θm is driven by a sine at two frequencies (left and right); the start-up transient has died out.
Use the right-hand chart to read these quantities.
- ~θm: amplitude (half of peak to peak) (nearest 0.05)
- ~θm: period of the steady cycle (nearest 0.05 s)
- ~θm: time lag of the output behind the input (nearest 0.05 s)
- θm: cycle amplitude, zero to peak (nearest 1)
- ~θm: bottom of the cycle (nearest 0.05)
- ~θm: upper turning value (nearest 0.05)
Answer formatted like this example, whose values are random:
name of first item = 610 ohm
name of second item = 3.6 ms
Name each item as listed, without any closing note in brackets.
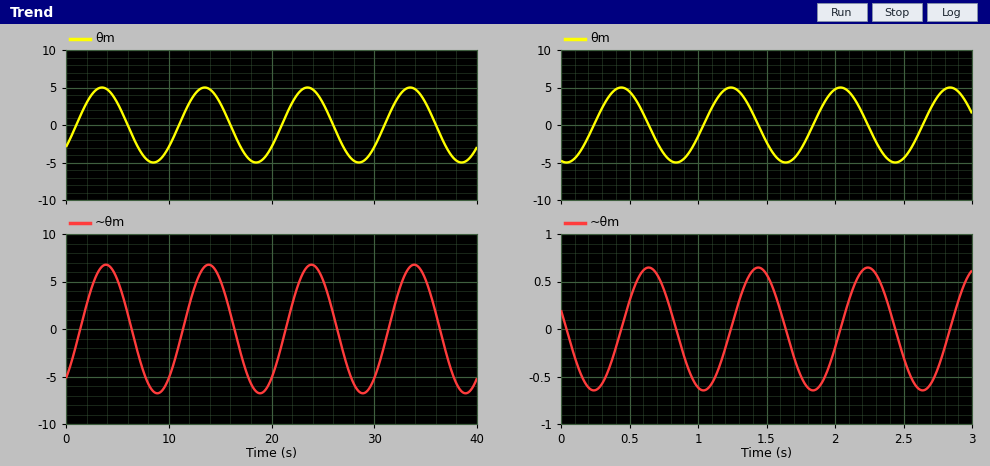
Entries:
~θm: amplitude (half of peak to peak) = 0.65
~θm: period of the steady cycle = 0.80 s
~θm: time lag of the output behind the input = 0.20 s
θm: cycle amplitude, zero to peak = 5
~θm: bottom of the cycle = -0.65
~θm: upper turning value = 0.65
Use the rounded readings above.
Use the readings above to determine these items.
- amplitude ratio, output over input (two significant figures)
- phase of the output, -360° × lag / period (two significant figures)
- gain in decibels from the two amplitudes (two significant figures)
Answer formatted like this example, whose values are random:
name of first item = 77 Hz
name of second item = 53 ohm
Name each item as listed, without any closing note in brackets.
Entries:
amplitude ratio, output over input = 0.13
phase of the output, -360° × lag / period = -90°
gain in decibels from the two amplitudes = -18 dB
